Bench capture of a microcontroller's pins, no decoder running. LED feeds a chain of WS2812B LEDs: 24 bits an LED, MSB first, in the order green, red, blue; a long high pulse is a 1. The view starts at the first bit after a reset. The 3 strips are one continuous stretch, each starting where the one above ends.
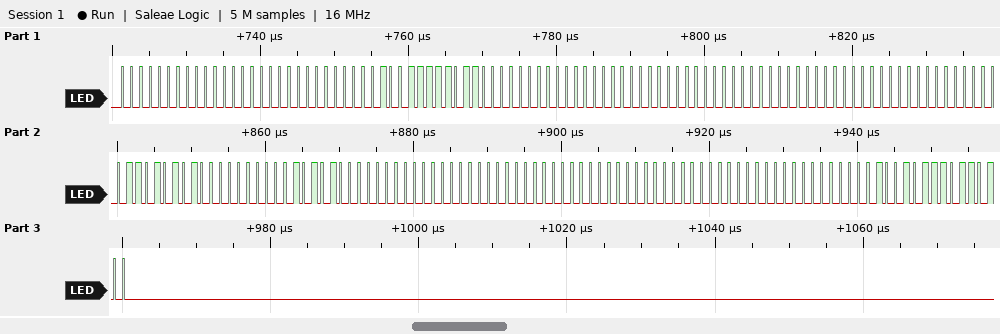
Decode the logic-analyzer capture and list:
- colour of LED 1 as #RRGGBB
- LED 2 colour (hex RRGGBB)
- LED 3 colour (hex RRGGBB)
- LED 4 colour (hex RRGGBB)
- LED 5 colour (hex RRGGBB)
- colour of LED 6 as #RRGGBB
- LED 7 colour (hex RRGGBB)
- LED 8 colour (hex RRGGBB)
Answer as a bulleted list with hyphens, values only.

- #000000
- #F60900
- #000000
- #000000
- #00D52A
- #000000
- #000000
- #4B00B4
